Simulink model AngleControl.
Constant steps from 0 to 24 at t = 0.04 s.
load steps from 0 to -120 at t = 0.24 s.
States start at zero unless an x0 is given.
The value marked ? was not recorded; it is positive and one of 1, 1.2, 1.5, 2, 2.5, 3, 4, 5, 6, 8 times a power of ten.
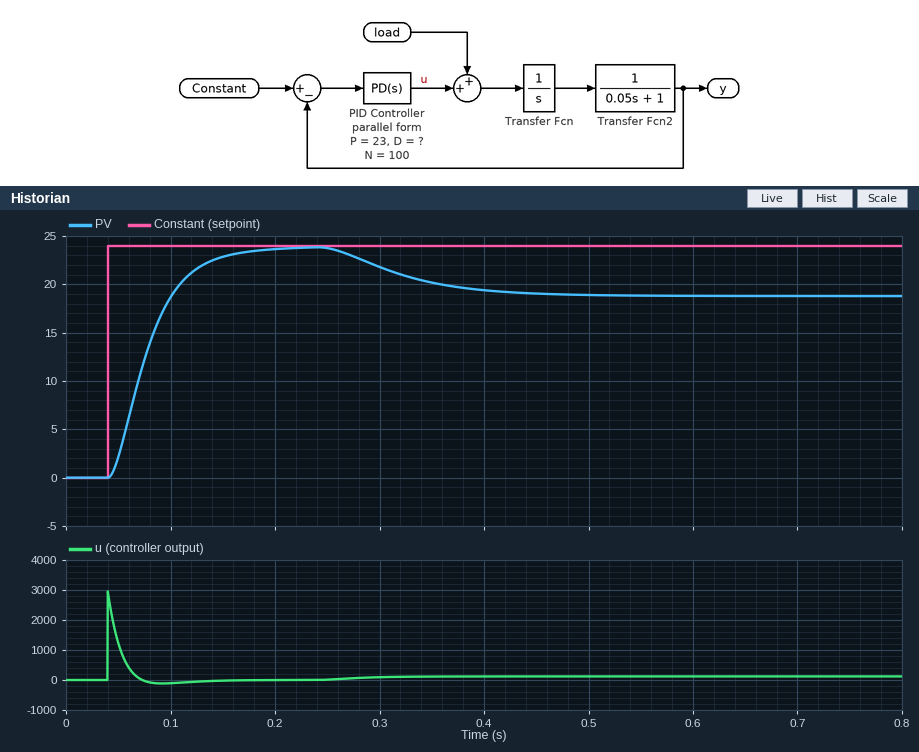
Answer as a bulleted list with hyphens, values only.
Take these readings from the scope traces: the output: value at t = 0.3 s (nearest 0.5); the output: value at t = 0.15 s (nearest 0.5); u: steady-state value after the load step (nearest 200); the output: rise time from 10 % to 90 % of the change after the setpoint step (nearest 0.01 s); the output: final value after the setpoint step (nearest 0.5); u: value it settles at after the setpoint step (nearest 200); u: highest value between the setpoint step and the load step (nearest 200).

- 22.0
- 23.0
- 200
- 0.07 s
- 24.0
- 0
- 3000
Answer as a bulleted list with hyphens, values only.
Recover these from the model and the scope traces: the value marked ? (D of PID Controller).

- 1
